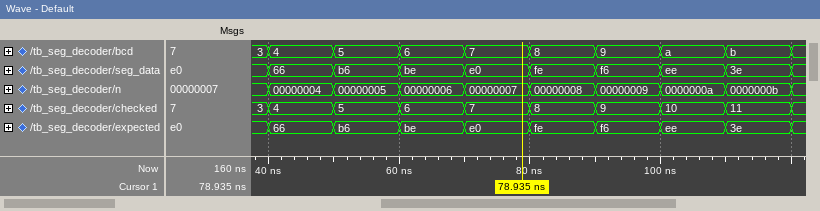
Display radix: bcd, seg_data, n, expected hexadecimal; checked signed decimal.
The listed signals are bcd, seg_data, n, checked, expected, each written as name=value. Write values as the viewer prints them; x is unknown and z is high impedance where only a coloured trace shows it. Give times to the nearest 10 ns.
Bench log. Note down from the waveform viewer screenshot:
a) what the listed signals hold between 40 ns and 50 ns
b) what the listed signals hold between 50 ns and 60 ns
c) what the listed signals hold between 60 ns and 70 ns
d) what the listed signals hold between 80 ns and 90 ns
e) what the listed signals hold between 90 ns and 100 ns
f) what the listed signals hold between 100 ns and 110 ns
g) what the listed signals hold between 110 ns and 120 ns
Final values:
bcd=4, seg_data=66, n=00000004, checked=4, expected=66
bcd=5, seg_data=b6, n=00000005, checked=5, expected=b6
bcd=6, seg_data=be, n=00000006, checked=6, expected=be
bcd=8, seg_data=fe, n=00000008, checked=8, expected=fe
bcd=9, seg_data=f6, n=00000009, checked=9, expected=f6
bcd=a, seg_data=ee, n=0000000a, checked=10, expected=ee
bcd=b, seg_data=3e, n=0000000b, checked=11, expected=3e
